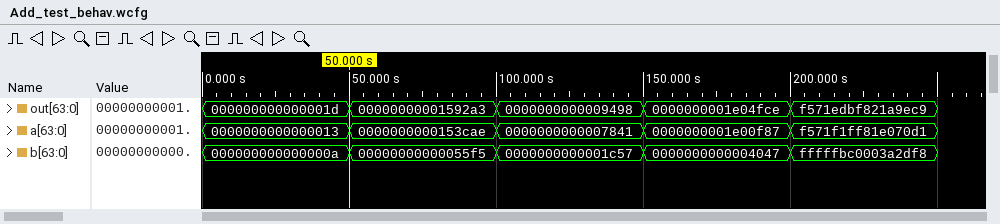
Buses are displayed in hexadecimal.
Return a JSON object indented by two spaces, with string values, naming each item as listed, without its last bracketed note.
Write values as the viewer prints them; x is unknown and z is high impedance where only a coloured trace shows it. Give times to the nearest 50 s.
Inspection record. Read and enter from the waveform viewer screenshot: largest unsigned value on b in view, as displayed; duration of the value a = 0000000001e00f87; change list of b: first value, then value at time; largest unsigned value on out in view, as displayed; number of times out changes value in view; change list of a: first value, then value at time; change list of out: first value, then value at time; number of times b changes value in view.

{
  "largest unsigned value on b in view, as displayed": "fffffbc0003a2df8",
  "duration of the value a = 0000000001e00f87": "50 s",
  "change list of b: first value, then value at time": "000000000000000a, 00000000000055f5 at 50 s, 0000000000001c57 at 100 s, 0000000000004047 at 150 s, fffffbc0003a2df8 at 200 s",
  "largest unsigned value on out in view, as displayed": "f571edbf821a9ec9",
  "number of times out changes value in view": "4",
  "change list of a: first value, then value at time": "0000000000000013, 0000000000153cae at 50 s, 0000000000007841 at 100 s, 0000000001e00f87 at 150 s, f571f1ff81e070d1 at 200 s",
  "change list of out: first value, then value at time": "000000000000001d, 00000000001592a3 at 50 s, 0000000000009498 at 100 s, 0000000001e04fce at 150 s, f571edbf821a9ec9 at 200 s",
  "number of times b changes value in view": "4"
}
